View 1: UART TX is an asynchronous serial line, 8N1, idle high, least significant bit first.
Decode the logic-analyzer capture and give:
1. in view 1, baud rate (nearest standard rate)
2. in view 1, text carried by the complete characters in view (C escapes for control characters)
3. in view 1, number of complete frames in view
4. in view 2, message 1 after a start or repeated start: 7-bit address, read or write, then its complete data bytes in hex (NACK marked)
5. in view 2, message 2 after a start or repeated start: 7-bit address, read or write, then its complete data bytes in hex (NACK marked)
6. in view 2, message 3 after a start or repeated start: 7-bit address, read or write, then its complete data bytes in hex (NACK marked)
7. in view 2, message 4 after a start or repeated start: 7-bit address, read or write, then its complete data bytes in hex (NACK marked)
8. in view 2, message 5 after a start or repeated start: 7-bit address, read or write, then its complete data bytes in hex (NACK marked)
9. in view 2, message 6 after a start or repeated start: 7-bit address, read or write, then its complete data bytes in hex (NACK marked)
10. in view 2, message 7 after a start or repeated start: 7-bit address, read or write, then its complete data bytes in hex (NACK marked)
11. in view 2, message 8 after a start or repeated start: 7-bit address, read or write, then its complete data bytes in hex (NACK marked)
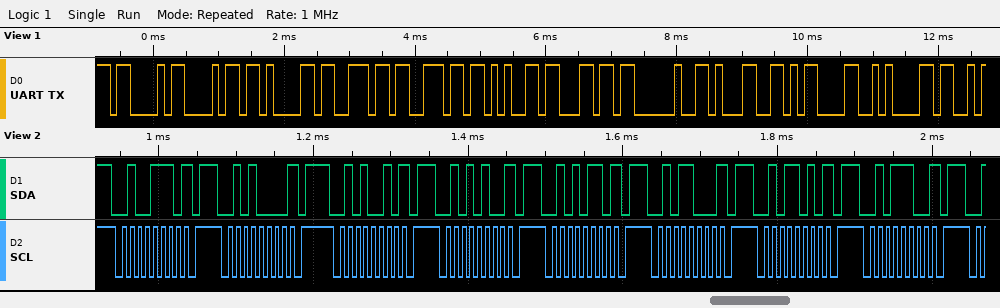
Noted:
9600 baud
"Channel 1\r\n"
11
0x27 write NACK
0x28 write NACK
0x29 write NACK
0x2A write NACK
0x2B write NACK
0x2C write NACK
0x2D write NACK
0x2E write NACK
